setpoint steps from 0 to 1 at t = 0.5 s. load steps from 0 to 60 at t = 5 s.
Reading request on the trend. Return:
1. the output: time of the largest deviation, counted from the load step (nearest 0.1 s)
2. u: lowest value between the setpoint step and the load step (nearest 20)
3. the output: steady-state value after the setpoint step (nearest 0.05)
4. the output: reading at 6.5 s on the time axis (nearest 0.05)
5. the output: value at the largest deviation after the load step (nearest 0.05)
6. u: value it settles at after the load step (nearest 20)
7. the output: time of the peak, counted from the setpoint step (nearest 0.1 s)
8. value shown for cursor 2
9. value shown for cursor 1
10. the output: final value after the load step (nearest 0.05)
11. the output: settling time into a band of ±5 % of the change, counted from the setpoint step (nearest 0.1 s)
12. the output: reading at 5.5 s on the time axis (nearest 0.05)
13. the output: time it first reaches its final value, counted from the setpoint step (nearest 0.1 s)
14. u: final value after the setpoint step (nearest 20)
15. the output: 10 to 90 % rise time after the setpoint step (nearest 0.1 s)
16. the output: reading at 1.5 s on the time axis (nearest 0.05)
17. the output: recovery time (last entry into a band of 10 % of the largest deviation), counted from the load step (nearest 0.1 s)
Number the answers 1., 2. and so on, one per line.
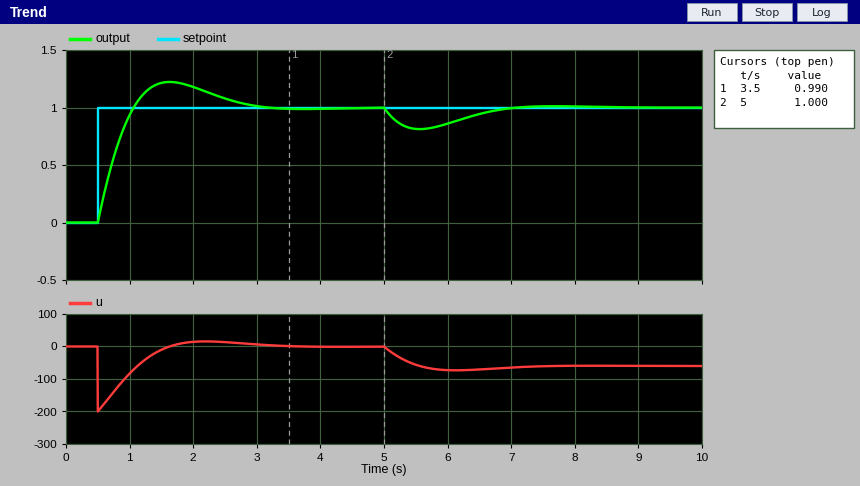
1. 0.6 s
2. -200
3. 1.00
4. 0.95
5. 0.80
6. -60
7. 1.1 s
8. 1.000
9. 0.990
10. 1.00
11. 2.2 s
12. 0.80
13. 0.6 s
14. 0
15. 0.4 s
16. 1.20
17. 1.8 s
